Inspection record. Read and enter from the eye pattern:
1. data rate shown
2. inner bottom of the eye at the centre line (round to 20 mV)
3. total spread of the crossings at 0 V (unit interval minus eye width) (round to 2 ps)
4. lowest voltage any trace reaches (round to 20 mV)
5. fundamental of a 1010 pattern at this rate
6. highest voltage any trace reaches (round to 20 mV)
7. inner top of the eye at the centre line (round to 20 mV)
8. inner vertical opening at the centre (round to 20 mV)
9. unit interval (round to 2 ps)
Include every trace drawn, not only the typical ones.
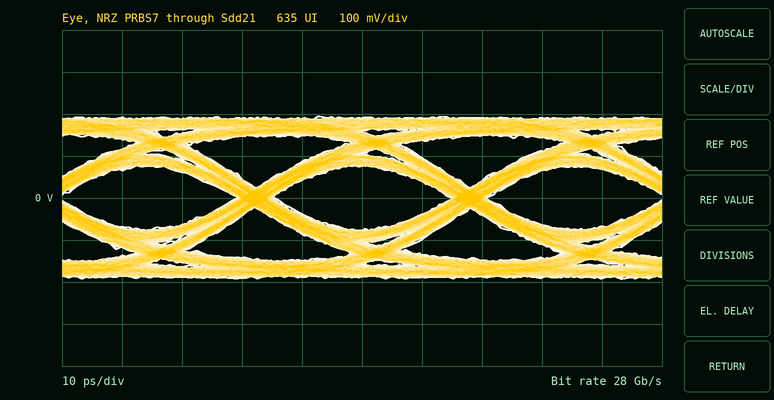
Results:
28 Gb/s
-80 mV
6 ps
-200 mV
14 GHz
200 mV
80 mV
160 mV
36 ps
